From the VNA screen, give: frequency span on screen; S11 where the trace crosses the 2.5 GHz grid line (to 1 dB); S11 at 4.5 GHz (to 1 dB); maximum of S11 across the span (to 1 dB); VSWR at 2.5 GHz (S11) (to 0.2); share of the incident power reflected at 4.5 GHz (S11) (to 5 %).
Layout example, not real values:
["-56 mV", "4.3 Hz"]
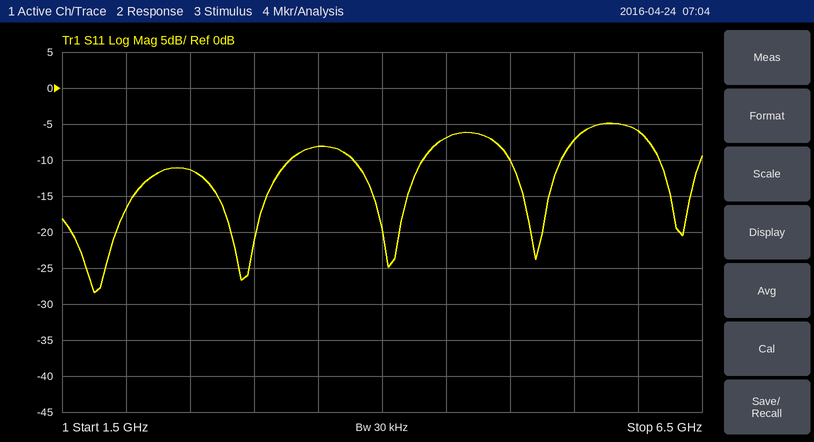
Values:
["5 GHz", "-11 dB", "-7 dB", "-5 dB", "1.8", "20 %"]
